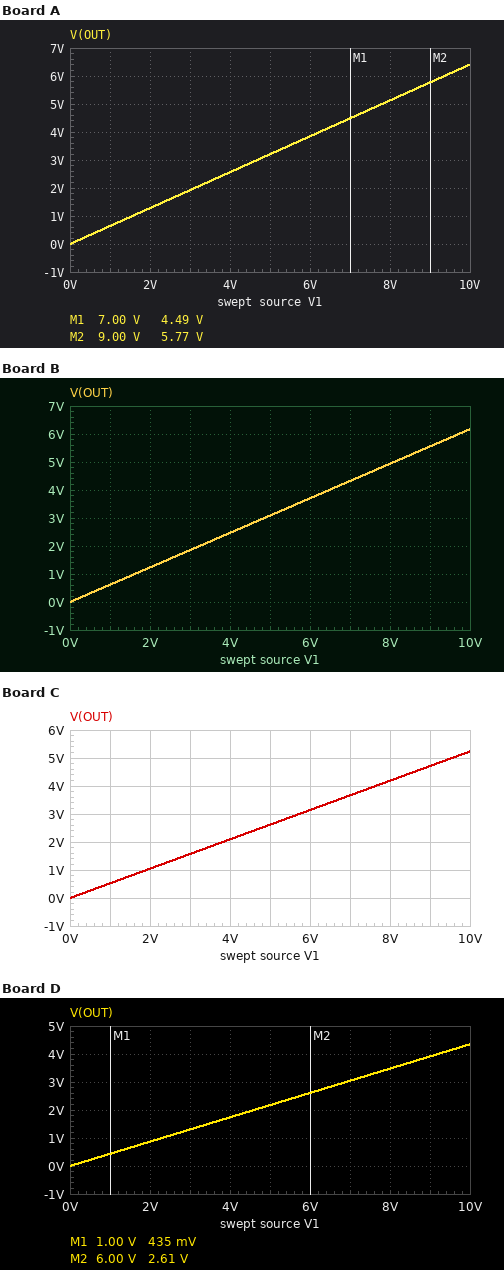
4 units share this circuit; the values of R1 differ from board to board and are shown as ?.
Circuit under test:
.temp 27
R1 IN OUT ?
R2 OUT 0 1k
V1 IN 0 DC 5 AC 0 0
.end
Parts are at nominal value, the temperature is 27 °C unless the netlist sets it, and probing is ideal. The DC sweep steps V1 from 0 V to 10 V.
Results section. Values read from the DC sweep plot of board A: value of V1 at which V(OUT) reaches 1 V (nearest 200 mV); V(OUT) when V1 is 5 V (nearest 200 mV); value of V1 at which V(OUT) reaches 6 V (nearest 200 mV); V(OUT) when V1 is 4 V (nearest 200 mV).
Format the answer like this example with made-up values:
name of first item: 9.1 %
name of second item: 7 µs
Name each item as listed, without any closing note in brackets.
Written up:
value of V1 at which V(OUT) reaches 1 V: 1.6 V
V(OUT) when V1 is 5 V: 3.2 V
value of V1 at which V(OUT) reaches 6 V: 9.4 V
V(OUT) when V1 is 4 V: 2.6 V
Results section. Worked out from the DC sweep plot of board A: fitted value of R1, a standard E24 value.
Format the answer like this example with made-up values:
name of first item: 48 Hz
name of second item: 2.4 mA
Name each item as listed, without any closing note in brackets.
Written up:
fitted value of R1, a standard E24 value: 560 Ω
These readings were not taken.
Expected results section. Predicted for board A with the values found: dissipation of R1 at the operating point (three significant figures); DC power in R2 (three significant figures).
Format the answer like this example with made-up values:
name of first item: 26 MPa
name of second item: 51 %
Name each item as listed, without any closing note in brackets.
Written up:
dissipation of R1 at the operating point: 5.75 mW
DC power in R2: 10.3 mW
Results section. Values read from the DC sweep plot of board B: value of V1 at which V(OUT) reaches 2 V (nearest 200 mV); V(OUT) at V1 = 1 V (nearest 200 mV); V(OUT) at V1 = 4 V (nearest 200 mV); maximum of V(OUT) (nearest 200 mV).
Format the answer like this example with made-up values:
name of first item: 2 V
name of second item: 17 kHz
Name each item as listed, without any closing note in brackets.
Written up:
value of V1 at which V(OUT) reaches 2 V: 3.2 V
V(OUT) at V1 = 1 V: 600 mV
V(OUT) at V1 = 4 V: 2.4 V
maximum of V(OUT): 6.2 V
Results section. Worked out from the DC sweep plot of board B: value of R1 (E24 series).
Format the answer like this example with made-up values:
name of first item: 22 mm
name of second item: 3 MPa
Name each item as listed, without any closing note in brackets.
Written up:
value of R1: 620 Ω
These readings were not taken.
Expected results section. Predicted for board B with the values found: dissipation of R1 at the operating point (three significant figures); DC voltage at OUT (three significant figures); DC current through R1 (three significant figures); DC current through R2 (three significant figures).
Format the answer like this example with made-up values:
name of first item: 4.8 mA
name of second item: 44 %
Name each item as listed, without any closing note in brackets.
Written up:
dissipation of R1 at the operating point: 5.91 mW
DC voltage at OUT: 3.09 V
DC current through R1: 3.09 mA
DC current through R2: 3.09 mA
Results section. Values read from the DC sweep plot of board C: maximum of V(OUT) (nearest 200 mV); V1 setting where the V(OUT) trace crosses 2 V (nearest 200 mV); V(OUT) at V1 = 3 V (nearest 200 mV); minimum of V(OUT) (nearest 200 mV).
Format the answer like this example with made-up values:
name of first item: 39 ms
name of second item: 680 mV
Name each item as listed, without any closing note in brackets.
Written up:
maximum of V(OUT): 5.2 V
V1 setting where the V(OUT) trace crosses 2 V: 3.8 V
V(OUT) at V1 = 3 V: 1.6 V
minimum of V(OUT): 0 V
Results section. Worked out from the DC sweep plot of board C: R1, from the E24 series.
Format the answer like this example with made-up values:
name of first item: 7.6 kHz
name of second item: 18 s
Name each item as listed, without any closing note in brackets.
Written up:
R1, from the E24 series: 910 Ω
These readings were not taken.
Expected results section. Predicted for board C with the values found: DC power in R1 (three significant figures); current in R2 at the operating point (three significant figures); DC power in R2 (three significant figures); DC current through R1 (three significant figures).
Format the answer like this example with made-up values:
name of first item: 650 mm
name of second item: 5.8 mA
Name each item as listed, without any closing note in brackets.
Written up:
DC power in R1: 6.24 mW
current in R2 at the operating point: 2.62 mA
DC power in R2: 6.85 mW
DC current through R1: 2.62 mA
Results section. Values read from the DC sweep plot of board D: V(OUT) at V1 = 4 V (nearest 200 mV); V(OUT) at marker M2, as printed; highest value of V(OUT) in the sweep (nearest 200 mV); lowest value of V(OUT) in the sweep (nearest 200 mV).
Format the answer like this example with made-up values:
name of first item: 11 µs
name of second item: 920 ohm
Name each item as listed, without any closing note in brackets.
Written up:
V(OUT) at V1 = 4 V: 1.8 V
V(OUT) at marker M2, as printed: 2.61 V
highest value of V(OUT) in the sweep: 4.4 V
lowest value of V(OUT) in the sweep: 0 V
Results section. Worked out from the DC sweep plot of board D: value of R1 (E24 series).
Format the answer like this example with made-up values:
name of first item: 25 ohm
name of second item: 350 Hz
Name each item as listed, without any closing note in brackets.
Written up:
value of R1: 1.3 kΩ
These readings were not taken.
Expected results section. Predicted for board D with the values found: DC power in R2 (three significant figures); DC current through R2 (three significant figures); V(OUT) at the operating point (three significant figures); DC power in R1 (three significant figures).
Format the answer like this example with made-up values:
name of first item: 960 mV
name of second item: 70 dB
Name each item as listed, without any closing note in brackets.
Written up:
DC power in R2: 4.73 mW
DC current through R2: 2.17 mA
V(OUT) at the operating point: 2.17 V
DC power in R1: 6.14 mW
